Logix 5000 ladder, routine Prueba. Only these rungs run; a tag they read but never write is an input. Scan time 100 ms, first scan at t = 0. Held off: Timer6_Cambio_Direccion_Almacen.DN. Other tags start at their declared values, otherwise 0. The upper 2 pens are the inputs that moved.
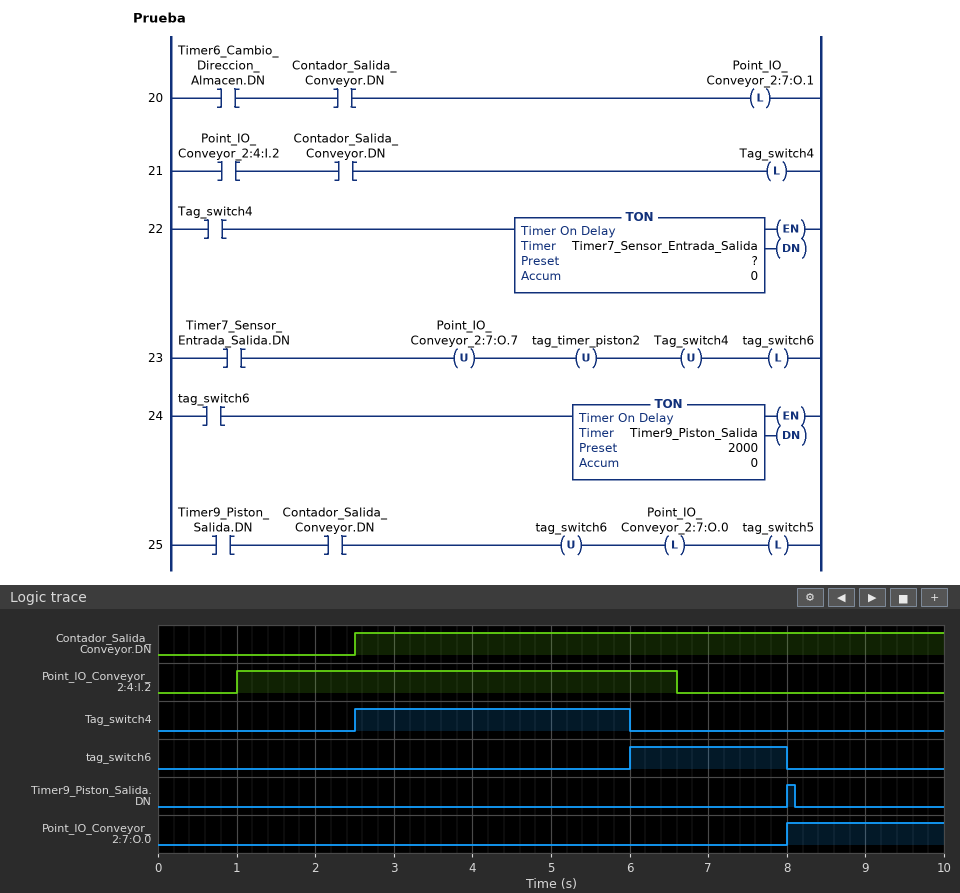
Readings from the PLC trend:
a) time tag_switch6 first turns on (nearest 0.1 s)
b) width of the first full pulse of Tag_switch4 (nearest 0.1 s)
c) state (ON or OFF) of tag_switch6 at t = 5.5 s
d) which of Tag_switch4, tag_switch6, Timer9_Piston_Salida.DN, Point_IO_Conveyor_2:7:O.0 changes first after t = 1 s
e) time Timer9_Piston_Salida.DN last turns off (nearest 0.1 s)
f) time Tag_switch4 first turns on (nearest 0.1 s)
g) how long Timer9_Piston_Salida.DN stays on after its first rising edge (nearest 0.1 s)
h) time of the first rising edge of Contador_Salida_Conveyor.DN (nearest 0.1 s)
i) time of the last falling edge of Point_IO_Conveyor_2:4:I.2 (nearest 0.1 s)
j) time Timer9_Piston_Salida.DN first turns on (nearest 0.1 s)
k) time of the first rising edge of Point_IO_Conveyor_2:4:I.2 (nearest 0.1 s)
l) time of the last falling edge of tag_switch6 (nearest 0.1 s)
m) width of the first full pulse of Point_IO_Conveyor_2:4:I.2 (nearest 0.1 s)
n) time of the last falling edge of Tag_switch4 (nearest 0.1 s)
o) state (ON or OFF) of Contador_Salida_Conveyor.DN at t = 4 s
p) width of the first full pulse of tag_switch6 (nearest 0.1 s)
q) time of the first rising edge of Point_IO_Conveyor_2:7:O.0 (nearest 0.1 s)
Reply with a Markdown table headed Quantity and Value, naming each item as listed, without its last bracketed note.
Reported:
| Quantity | Value |
|---|---|
| time tag_switch6 first turns on | 6.0 s |
| width of the first full pulse of Tag_switch4 | 3.5 s |
| state (ON or OFF) of tag_switch6 at t = 5.5 s | OFF |
| which of Tag_switch4, tag_switch6, Timer9_Piston_Salida.DN, Point_IO_Conveyor_2:7:O.0 changes first after t = 1 s | Tag_switch4 |
| time Timer9_Piston_Salida.DN last turns off | 8.1 s |
| time Tag_switch4 first turns on | 2.5 s |
| how long Timer9_Piston_Salida.DN stays on after its first rising edge | 0.1 s |
| time of the first rising edge of Contador_Salida_Conveyor.DN | 2.5 s |
| time of the last falling edge of Point_IO_Conveyor_2:4:I.2 | 6.6 s |
| time Timer9_Piston_Salida.DN first turns on | 8.0 s |
| time of the first rising edge of Point_IO_Conveyor_2:4:I.2 | 1.0 s |
| time of the last falling edge of tag_switch6 | 8.0 s |
| width of the first full pulse of Point_IO_Conveyor_2:4:I.2 | 5.6 s |
| time of the last falling edge of Tag_switch4 | 6.0 s |
| state (ON or OFF) of Contador_Salida_Conveyor.DN at t = 4 s | ON |
| width of the first full pulse of tag_switch6 | 2.0 s |
| time of the first rising edge of Point_IO_Conveyor_2:7:O.0 | 8.0 s |
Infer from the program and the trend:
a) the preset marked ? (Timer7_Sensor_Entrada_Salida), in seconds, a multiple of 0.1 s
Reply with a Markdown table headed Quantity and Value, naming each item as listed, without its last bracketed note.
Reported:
| Quantity | Value |
|---|---|
| the preset marked ? (Timer7_Sensor_Entrada_Salida), in seconds, a multiple of 0.1 s | 3.5 s |
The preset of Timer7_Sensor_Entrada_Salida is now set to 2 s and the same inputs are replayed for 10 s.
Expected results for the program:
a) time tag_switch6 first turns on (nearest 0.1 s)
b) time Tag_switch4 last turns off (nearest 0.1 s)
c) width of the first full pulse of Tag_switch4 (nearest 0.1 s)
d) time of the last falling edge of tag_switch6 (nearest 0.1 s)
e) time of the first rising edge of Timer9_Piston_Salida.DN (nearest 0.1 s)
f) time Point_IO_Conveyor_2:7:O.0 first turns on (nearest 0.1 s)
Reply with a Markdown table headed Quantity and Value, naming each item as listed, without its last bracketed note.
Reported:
| Quantity | Value |
|---|---|
| time tag_switch6 first turns on | 4.5 s |
| time Tag_switch4 last turns off | 4.5 s |
| width of the first full pulse of Tag_switch4 | 2.0 s |
| time of the last falling edge of tag_switch6 | 6.5 s |
| time of the first rising edge of Timer9_Piston_Salida.DN | 6.5 s |
| time Point_IO_Conveyor_2:7:O.0 first turns on | 6.5 s |
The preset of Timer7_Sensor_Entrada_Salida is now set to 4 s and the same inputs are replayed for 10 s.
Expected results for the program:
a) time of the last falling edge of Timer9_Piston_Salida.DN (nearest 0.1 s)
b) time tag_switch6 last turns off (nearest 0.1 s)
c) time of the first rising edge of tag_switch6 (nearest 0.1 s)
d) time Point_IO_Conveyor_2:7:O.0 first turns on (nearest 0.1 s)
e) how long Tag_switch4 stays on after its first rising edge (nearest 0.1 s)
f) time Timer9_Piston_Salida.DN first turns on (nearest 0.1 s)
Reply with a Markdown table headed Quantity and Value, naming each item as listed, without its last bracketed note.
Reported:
| Quantity | Value |
|---|---|
| time of the last falling edge of Timer9_Piston_Salida.DN | 8.6 s |
| time tag_switch6 last turns off | 8.5 s |
| time of the first rising edge of tag_switch6 | 6.5 s |
| time Point_IO_Conveyor_2:7:O.0 first turns on | 8.5 s |
| how long Tag_switch4 stays on after its first rising edge | 4.0 s |
| time Timer9_Piston_Salida.DN first turns on | 8.5 s |
